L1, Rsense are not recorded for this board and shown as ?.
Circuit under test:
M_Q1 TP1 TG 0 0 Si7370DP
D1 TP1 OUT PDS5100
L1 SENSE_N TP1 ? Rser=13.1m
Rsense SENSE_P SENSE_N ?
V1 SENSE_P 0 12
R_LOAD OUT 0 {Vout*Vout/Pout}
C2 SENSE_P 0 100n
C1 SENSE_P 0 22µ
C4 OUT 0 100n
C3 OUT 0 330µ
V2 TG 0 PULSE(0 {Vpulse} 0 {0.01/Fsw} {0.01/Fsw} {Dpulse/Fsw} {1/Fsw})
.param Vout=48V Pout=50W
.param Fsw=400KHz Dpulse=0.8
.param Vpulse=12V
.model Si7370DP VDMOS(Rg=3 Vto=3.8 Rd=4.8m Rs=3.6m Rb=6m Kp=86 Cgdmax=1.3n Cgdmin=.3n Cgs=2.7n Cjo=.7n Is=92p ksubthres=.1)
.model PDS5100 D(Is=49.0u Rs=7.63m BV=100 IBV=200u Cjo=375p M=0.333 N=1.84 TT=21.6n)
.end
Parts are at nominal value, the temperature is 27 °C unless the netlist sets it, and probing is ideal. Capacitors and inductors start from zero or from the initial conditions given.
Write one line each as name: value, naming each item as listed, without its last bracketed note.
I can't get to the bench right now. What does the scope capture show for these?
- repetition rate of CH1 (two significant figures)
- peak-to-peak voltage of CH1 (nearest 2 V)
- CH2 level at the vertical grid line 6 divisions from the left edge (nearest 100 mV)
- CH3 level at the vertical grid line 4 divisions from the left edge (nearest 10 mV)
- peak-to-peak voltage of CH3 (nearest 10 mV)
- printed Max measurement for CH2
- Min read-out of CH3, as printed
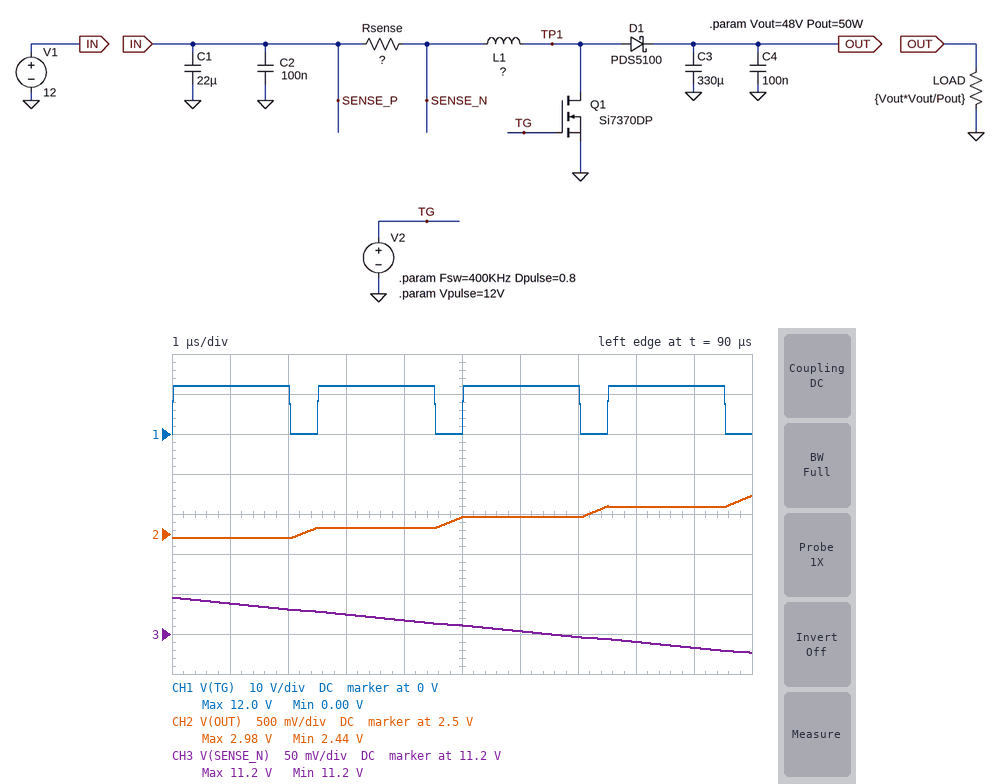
repetition rate of CH1: 400 kHz
peak-to-peak voltage of CH1: 12 V
CH2 level at the vertical grid line 6 divisions from the left edge: 2.7 V
CH3 level at the vertical grid line 4 divisions from the left edge: 11.22 V
peak-to-peak voltage of CH3: 70 mV
printed Max measurement for CH2: 2.98 V
Min read-out of CH3, as printed: 11.2 V
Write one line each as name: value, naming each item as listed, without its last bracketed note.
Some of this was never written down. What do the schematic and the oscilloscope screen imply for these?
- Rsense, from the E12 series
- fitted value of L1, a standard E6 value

Rsense, from the E12 series: 8.2 mΩ
fitted value of L1, a standard E6 value: 10 µH
